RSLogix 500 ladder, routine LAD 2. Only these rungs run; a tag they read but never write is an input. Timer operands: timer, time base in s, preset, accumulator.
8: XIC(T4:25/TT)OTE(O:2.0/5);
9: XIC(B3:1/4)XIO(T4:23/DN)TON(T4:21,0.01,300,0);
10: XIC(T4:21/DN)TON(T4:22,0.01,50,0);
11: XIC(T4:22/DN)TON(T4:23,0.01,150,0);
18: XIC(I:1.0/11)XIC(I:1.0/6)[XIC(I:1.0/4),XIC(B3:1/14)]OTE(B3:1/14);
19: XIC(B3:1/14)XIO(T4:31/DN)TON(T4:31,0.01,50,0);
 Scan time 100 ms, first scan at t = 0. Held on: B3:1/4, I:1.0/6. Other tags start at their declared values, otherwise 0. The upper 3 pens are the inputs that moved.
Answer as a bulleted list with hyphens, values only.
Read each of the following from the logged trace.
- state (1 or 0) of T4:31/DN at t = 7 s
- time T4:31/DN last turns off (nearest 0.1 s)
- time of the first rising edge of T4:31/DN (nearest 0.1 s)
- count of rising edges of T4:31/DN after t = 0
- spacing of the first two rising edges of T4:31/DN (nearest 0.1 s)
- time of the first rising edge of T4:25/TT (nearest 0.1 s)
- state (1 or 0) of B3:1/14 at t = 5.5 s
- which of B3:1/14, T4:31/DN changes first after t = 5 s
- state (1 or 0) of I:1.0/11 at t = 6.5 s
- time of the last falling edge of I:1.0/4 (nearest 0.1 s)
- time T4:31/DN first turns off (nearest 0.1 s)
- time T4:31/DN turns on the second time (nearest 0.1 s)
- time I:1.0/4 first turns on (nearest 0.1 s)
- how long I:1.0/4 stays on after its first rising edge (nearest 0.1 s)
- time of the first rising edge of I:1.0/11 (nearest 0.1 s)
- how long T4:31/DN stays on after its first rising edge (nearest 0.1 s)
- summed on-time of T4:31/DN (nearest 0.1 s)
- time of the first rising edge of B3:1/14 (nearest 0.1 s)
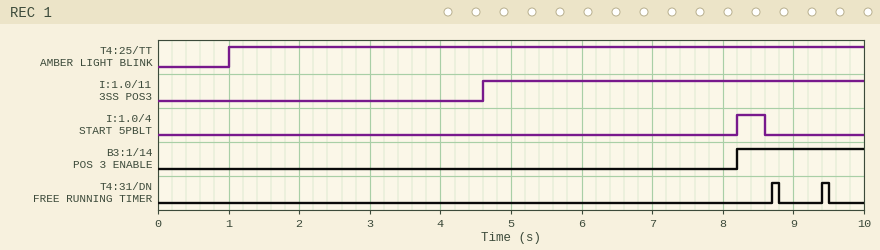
- 0
- 9.5 s
- 8.7 s
- 2
- 0.7 s
- 1.0 s
- 0
- B3:1/14
- 1
- 8.6 s
- 8.8 s
- 9.4 s
- 8.2 s
- 0.4 s
- 4.6 s
- 0.1 s
- 0.2 s
- 8.2 s
